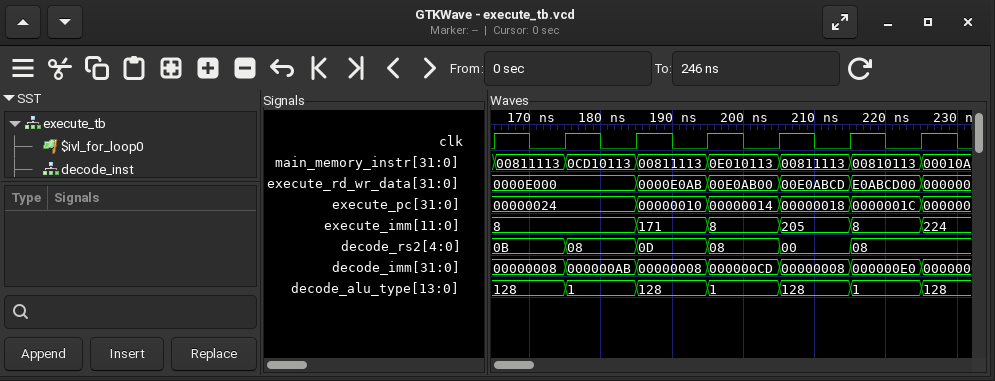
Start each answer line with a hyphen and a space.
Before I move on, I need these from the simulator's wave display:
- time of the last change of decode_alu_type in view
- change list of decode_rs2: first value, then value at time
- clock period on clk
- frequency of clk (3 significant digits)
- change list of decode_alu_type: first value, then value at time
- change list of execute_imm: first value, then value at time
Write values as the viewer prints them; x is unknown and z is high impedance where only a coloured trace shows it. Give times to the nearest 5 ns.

- 225 ns
- 0B, 08 at 175 ns, 0D at 185 ns, 08 at 195 ns, 00 at 205 ns, 08 at 215 ns
- 10 ns
- 100 MHz
- 128, 1 at 175 ns, 128 at 185 ns, 1 at 195 ns, 128 at 205 ns, 1 at 215 ns, 128 at 225 ns
- 8, 171 at 185 ns, 8 at 195 ns, 205 at 205 ns, 8 at 215 ns, 224 at 225 ns
